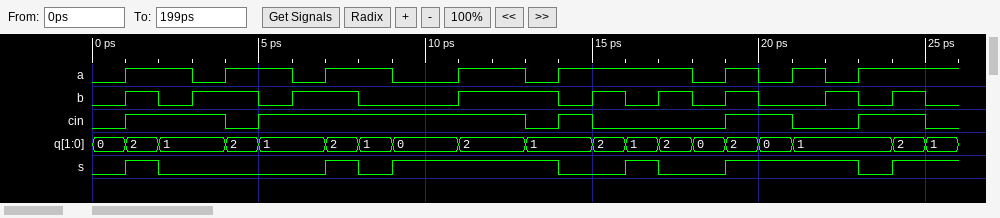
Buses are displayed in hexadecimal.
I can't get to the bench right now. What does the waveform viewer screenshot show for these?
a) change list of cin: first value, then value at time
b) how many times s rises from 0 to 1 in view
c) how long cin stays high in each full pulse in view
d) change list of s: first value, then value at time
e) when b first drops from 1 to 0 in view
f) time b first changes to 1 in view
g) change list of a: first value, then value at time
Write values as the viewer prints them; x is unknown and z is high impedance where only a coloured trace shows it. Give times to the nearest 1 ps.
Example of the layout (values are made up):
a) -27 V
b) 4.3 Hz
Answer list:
a) 0, 1 at 1 ps, 0 at 4 ps, 1 at 5 ps, 0 at 13 ps, 1 at 14 ps, 0 at 15 ps, 1 at 19 ps, 0 at 21 ps, 1 at 23 ps, 0 at 25 ps
b) 6
c) 3 ps, 8 ps, 1 ps, 2 ps, 2 ps
d) 0, 1 at 1 ps, 0 at 2 ps, 1 at 7 ps, 0 at 8 ps, 1 at 9 ps, 0 at 14 ps, 1 at 16 ps, 0 at 17 ps, 1 at 19 ps, 0 at 23 ps, 1 at 24 ps
e) 2 ps
f) 1 ps
g) 0, 1 at 1 ps, 0 at 3 ps, 1 at 4 ps, 0 at 6 ps, 1 at 7 ps, 0 at 9 ps, 1 at 11 ps, 0 at 13 ps, 1 at 14 ps, 0 at 18 ps, 1 at 19 ps, 0 at 20 ps, 1 at 21 ps, 0 at 22 ps, 1 at 23 ps
